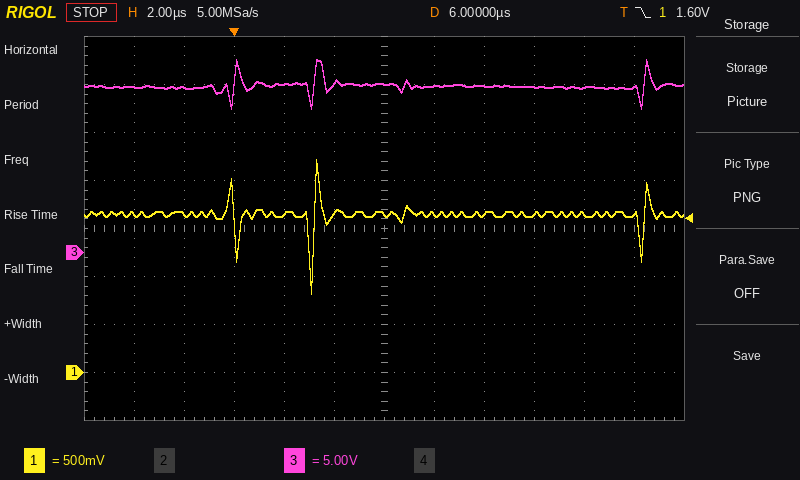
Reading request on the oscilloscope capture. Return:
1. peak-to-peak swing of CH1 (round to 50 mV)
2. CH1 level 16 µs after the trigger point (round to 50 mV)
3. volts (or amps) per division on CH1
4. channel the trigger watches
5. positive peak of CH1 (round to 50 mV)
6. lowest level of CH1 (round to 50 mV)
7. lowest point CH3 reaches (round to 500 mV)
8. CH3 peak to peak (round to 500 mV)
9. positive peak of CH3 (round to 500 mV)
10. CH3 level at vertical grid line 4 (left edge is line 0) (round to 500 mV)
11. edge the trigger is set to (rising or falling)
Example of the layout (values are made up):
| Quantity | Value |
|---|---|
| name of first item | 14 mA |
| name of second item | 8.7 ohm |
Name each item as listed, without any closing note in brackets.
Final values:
| Quantity | Value |
|---|---|
| peak-to-peak swing of CH1 | 1.40 V |
| CH1 level 16 µs after the trigger point | 1.65 V |
| volts (or amps) per division on CH1 | 500 mV |
| channel the trigger watches | CH1 |
| positive peak of CH1 | 2.20 V |
| lowest level of CH1 | 800 mV |
| lowest point CH3 reaches | 15.0 V |
| CH3 peak to peak | 5.0 V |
| positive peak of CH3 | 20.0 V |
| CH3 level at vertical grid line 4 (left edge is line 0) | 17.5 V |
| edge the trigger is set to | falling |
